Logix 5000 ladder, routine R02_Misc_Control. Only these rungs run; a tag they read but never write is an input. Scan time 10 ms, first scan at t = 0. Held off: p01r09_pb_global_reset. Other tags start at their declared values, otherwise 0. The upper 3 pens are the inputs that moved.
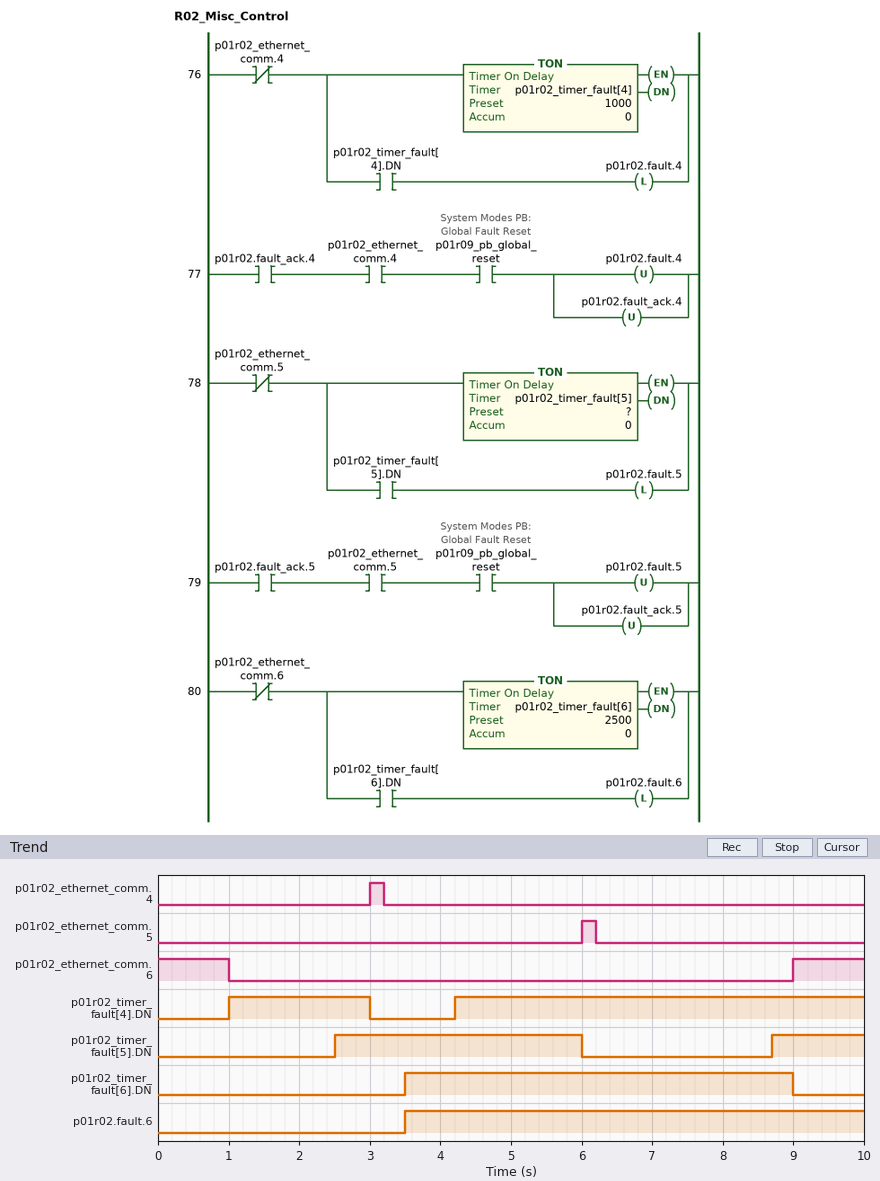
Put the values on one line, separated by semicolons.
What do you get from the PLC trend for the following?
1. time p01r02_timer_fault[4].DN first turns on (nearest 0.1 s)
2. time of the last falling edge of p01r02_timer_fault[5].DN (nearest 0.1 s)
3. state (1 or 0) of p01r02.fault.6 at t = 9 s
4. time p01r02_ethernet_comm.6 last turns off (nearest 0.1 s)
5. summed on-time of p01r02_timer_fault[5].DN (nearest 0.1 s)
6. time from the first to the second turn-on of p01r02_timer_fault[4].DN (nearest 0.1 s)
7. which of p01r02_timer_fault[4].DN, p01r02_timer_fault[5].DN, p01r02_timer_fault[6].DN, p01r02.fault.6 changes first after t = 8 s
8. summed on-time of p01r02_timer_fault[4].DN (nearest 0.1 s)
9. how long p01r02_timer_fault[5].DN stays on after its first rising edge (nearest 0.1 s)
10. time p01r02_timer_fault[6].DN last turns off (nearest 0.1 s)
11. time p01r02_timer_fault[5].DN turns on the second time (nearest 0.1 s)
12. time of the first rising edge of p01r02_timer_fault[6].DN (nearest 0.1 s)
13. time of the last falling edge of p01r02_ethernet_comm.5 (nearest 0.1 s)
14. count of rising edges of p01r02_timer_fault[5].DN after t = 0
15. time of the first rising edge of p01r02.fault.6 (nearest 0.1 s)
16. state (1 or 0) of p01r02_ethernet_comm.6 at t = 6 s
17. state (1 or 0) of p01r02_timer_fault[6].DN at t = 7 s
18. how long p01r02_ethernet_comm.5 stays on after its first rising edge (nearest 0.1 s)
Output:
1.0 s; 6.0 s; 1; 1.0 s; 4.8 s; 3.2 s; p01r02_timer_fault[5].DN; 7.8 s; 3.5 s; 9.0 s; 8.7 s; 3.5 s; 6.2 s; 2; 3.5 s; 0; 1; 0.2 s
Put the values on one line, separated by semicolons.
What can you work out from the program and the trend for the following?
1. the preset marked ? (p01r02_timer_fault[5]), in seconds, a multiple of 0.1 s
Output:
2.5 s
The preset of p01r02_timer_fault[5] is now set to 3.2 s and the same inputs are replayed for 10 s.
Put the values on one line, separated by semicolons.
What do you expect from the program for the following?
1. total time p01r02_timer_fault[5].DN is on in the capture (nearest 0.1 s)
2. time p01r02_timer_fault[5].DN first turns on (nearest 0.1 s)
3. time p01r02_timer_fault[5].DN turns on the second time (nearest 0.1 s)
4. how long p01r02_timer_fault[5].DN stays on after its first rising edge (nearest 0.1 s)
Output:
3.4 s; 3.2 s; 9.4 s; 2.8 s
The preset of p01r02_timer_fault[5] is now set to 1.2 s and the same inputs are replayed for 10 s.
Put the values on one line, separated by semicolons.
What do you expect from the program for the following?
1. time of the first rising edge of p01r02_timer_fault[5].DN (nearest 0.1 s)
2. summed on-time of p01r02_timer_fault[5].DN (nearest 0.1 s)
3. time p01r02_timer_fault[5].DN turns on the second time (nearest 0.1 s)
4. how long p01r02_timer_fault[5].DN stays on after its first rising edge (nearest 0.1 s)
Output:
1.2 s; 7.4 s; 7.4 s; 4.8 s
